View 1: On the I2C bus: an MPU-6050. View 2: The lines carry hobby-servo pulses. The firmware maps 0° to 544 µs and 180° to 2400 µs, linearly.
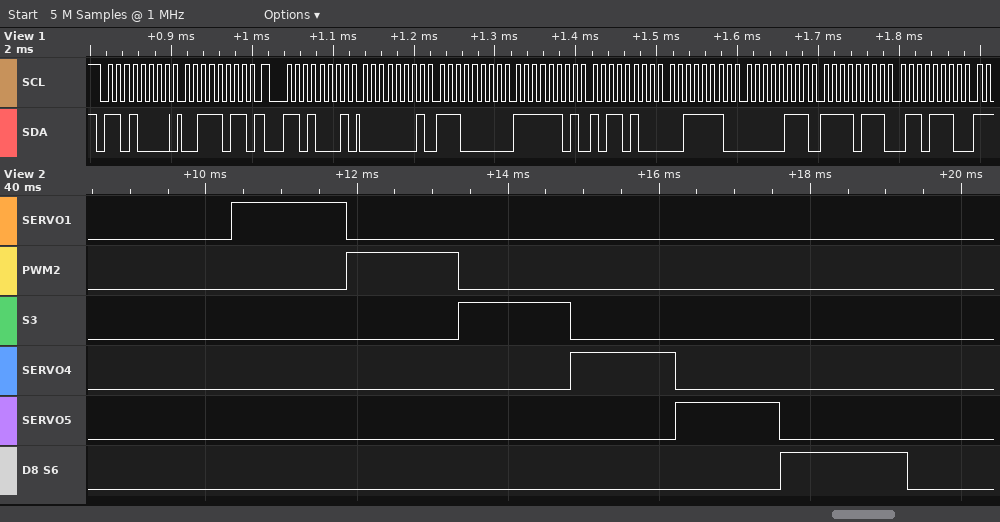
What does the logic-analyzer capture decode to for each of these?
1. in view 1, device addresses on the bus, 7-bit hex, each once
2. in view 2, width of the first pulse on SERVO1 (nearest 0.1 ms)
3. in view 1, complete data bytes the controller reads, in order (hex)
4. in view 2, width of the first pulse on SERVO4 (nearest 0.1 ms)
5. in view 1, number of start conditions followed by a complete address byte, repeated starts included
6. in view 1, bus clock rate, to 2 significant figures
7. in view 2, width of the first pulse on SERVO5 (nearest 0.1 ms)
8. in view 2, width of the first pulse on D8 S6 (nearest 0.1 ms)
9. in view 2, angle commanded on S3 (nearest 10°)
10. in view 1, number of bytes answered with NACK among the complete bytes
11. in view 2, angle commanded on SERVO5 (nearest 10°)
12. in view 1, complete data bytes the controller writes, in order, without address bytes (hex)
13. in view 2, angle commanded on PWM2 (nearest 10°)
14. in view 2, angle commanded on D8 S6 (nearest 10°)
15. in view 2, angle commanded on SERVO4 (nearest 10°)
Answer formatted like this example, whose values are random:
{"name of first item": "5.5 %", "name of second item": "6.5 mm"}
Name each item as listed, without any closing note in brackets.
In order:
{"in view 1, device addresses on the bus, 7-bit hex, each once": "0x68", "in view 2, width of the first pulse on SERVO1": "1.5 ms", "in view 1, complete data bytes the controller reads, in order": "01 E0 FD B4 3E 07 F7 6E", "in view 2, width of the first pulse on SERVO4": "1.4 ms", "in view 1, number of start conditions followed by a complete address byte, repeated starts included": "2", "in view 1, bus clock rate, to 2 significant figures": "100 kHz", "in view 2, width of the first pulse on SERVO5": "1.4 ms", "in view 2, width of the first pulse on D8 S6": "1.7 ms", "in view 2, angle commanded on S3": "90°", "in view 1, number of bytes answered with NACK among the complete bytes": "0", "in view 2, angle commanded on SERVO5": "80°", "in view 1, complete data bytes the controller writes, in order, without address bytes": "3B", "in view 2, angle commanded on PWM2": "90°", "in view 2, angle commanded on D8 S6": "110°", "in view 2, angle commanded on SERVO4": "80°"}
